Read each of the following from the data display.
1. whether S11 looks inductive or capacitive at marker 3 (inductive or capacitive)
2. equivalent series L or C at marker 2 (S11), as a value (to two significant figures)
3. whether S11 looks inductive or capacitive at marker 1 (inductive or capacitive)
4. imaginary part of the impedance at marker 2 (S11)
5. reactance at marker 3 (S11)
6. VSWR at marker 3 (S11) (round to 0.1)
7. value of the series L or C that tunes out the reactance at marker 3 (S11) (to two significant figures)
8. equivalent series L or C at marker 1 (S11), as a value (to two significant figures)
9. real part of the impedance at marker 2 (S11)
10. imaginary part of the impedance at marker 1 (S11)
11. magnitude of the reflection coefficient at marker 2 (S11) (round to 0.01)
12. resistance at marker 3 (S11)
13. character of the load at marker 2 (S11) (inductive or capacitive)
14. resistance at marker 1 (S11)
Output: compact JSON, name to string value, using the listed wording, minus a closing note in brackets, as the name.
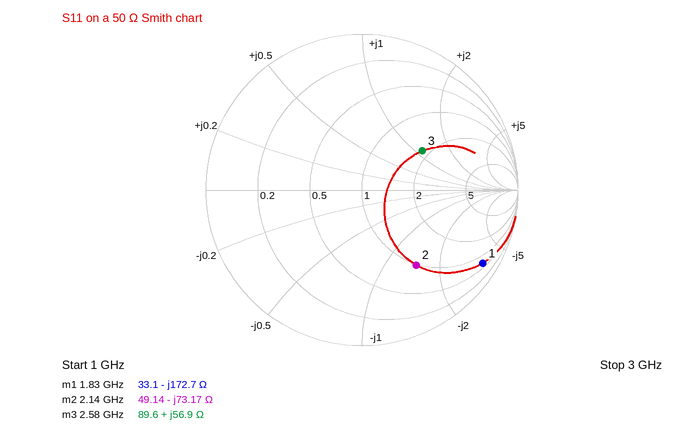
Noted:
{"whether S11 looks inductive or capacitive at marker 3": "inductive", "equivalent series L or C at marker 2 (S11), as a value": "1.0 pF", "whether S11 looks inductive or capacitive at marker 1": "capacitive", "imaginary part of the impedance at marker 2": "-73.17 Ω", "reactance at marker 3": "+56.9 Ω", "VSWR at marker 3 (S11)": "2.7", "value of the series L or C that tunes out the reactance at marker 3 (S11)": "1.1 pF", "equivalent series L or C at marker 1 (S11), as a value": "500 fF", "real part of the impedance at marker 2": "49.14 Ω", "imaginary part of the impedance at marker 1": "-172.7 Ω", "magnitude of the reflection coefficient at marker 2 (S11)": "0.59", "resistance at marker 3": "89.6 Ω", "character of the load at marker 2 (S11)": "capacitive", "resistance at marker 1": "33.1 Ω"}
